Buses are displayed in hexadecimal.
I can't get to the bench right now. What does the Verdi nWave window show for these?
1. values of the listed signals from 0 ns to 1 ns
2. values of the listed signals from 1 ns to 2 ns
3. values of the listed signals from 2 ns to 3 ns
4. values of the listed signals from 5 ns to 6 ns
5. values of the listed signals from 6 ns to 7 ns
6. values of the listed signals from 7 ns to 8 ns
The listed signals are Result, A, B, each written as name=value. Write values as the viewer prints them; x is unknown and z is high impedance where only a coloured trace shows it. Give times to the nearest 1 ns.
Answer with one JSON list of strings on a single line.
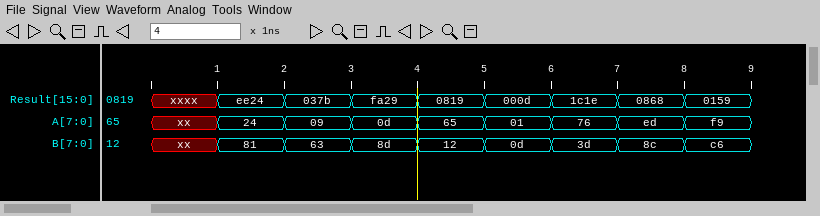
["Result=xxxx, A=xx, B=xx", "Result=ee24, A=24, B=81", "Result=037b, A=09, B=63", "Result=000d, A=01, B=0d", "Result=1c1e, A=76, B=3d", "Result=0868, A=ed, B=8c"]
